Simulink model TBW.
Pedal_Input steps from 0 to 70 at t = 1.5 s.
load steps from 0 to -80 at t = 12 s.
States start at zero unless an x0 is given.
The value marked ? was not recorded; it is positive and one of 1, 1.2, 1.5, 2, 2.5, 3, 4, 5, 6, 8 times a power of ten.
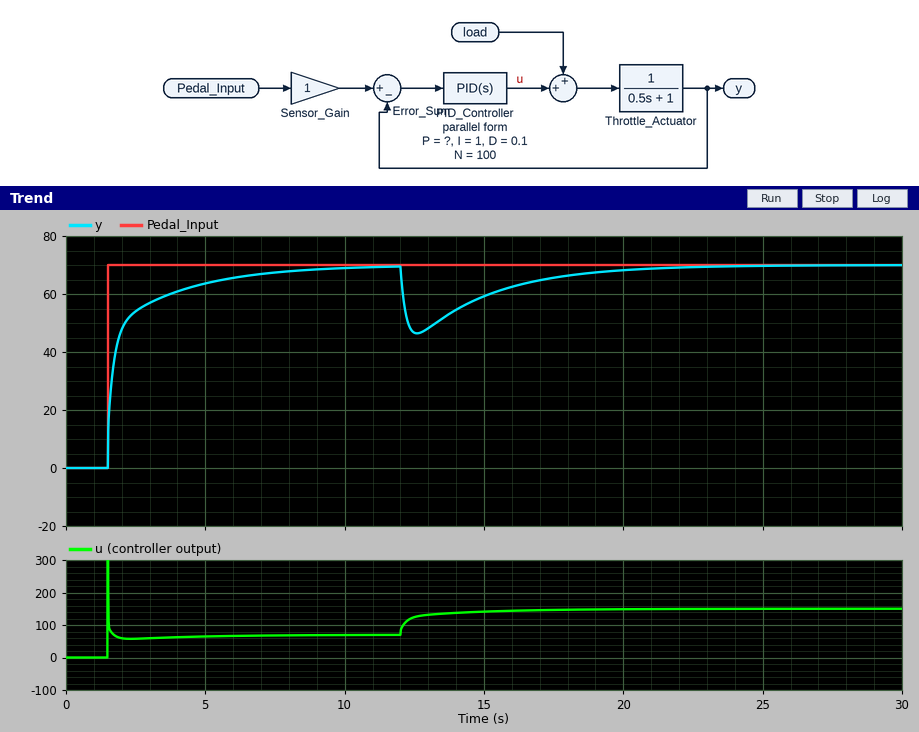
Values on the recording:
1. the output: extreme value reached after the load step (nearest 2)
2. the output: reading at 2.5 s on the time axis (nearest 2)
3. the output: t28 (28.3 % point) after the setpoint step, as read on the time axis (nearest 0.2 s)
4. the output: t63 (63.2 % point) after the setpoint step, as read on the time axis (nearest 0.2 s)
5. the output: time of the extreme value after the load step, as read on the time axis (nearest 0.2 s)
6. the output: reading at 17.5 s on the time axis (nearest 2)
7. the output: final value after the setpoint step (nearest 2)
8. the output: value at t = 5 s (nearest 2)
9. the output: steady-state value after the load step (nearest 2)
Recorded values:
46
54
1.6 s
1.8 s
12.6 s
66
70
64
70
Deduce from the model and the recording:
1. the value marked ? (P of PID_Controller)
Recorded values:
2
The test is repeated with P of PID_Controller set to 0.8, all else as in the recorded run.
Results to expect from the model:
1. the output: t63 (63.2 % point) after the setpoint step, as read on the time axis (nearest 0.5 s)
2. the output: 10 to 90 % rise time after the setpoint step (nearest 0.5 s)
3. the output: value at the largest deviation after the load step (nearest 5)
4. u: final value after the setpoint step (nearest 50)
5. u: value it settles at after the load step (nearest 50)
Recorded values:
2.5 s
2.5 s
35
50
150
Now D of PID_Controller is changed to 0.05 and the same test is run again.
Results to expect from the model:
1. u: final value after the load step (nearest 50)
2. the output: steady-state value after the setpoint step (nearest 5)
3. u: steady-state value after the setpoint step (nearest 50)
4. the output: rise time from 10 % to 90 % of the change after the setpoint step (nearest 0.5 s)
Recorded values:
150
70
50
3.0 s
